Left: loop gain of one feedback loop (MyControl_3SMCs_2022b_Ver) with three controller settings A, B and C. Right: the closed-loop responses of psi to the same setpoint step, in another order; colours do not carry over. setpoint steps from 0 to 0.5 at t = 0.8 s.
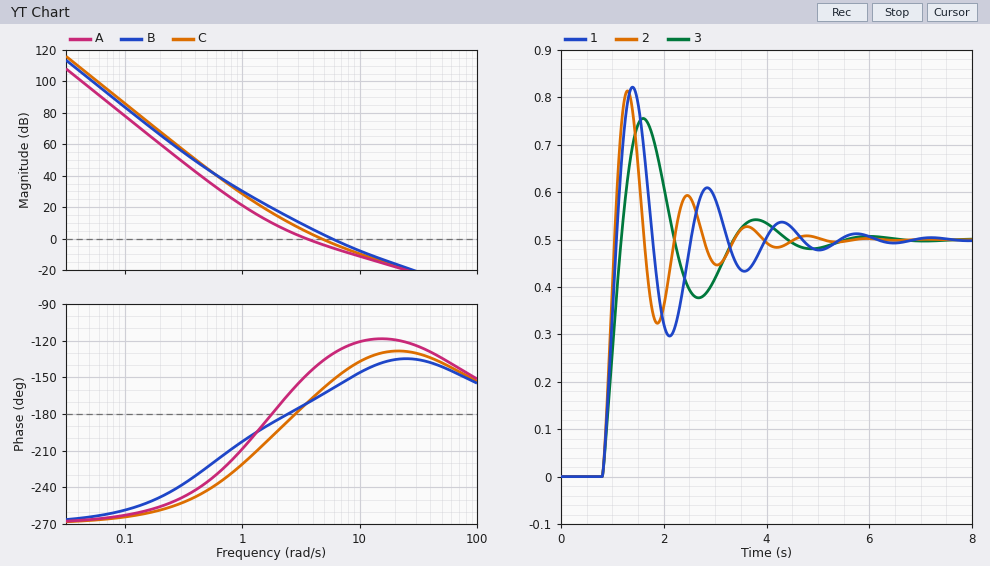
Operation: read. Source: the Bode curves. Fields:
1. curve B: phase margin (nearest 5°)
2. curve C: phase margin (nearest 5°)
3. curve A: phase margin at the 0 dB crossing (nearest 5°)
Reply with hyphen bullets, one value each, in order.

- 20°
- 20°
- 30°
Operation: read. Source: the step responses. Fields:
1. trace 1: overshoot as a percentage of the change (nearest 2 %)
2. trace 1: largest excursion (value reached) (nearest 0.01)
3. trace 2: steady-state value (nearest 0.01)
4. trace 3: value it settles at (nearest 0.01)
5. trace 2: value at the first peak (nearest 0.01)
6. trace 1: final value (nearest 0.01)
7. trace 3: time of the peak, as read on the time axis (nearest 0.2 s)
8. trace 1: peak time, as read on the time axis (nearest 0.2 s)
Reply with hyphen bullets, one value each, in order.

- 64 %
- 0.82
- 0.50
- 0.50
- 0.81
- 0.50
- 1.6 s
- 1.4 s
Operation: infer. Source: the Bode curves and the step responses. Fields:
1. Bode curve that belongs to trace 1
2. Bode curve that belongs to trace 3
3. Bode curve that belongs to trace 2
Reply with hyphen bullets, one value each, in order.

- C
- A
- B
